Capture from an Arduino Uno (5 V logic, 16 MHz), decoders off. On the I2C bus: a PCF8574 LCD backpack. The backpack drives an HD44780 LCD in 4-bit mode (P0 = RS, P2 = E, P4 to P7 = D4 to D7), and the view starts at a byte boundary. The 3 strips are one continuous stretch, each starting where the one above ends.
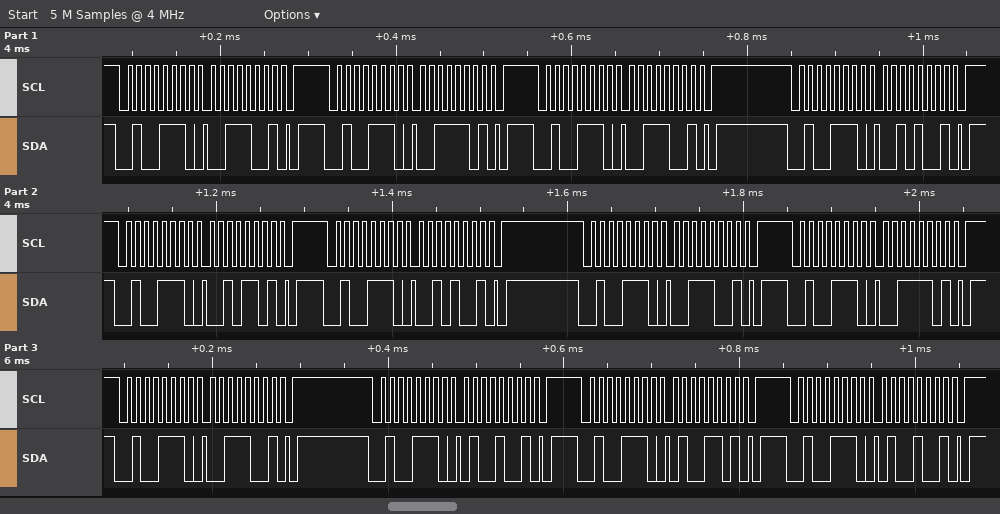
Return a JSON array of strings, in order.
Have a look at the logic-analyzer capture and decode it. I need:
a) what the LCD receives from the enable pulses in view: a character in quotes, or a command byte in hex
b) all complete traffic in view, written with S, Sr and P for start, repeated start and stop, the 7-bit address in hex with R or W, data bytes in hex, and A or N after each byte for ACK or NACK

["'2' '4'", "S 27W A 39 A P S 27W A 3D A P S 27W A 39 A P S 27W A 29 A P S 27W A 2D A P S 27W A 29 A P S 27W A 39 A P S 27W A 3D A P S 27W A 39 A P S 27W A 49 A P S 27W A 4D A P S 27W A 49 A P"]
